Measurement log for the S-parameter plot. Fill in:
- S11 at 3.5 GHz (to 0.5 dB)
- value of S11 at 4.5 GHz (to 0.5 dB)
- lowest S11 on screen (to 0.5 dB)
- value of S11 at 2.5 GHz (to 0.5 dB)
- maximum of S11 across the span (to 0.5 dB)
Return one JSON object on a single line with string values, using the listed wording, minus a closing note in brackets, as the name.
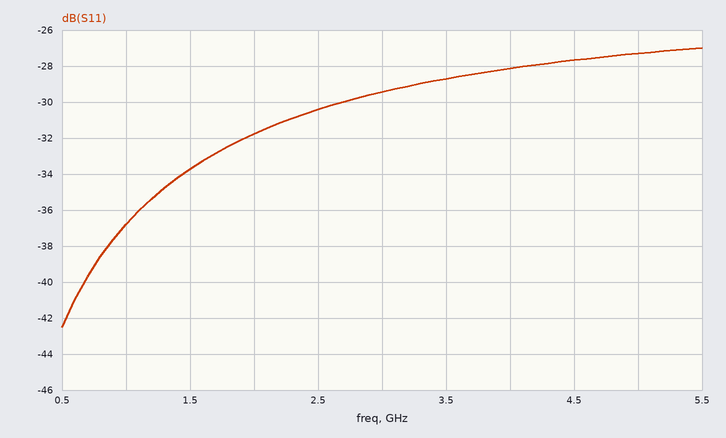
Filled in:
{"S11 at 3.5 GHz": "-28.5 dB", "value of S11 at 4.5 GHz": "-27.5 dB", "lowest S11 on screen": "-42.5 dB", "value of S11 at 2.5 GHz": "-30.5 dB", "maximum of S11 across the span": "-27.0 dB"}
